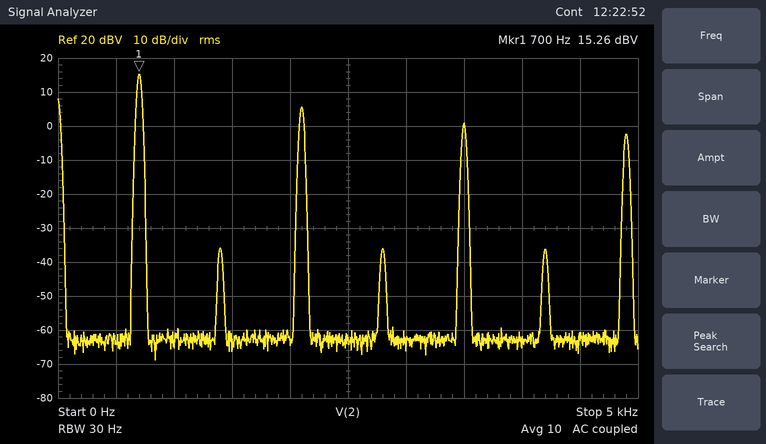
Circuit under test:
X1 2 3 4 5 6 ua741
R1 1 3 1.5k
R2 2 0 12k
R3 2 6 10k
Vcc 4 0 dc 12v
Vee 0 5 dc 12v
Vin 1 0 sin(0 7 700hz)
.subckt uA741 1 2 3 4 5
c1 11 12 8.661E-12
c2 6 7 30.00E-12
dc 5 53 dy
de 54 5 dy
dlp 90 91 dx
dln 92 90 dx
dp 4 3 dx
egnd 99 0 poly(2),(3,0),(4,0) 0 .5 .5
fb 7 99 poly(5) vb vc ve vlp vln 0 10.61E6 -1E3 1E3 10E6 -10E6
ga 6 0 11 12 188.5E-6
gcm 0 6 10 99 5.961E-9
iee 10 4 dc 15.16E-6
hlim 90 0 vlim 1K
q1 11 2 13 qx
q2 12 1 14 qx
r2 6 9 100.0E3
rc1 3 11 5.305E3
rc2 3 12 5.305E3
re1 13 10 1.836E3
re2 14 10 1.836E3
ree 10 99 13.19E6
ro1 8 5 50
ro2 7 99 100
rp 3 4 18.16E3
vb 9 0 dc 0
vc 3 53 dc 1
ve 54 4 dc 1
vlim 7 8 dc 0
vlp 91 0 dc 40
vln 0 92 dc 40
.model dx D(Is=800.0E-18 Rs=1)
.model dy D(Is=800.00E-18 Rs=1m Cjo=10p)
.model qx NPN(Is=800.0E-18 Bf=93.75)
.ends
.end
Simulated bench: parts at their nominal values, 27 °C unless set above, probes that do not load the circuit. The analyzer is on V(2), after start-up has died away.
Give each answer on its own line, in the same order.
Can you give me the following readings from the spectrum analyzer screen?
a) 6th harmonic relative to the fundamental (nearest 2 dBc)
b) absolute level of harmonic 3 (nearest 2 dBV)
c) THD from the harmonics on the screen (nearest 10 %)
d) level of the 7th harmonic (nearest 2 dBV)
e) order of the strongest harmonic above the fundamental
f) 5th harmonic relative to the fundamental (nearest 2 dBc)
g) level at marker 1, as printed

-52 dBc
6 dBV
40 %
-2 dBV
3
-14 dBc
15.26 dBV
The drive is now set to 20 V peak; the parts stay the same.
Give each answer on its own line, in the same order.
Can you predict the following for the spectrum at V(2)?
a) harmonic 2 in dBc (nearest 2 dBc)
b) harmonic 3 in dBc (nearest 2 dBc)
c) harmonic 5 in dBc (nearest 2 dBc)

2 dBc
0 dBc
-4 dBc
